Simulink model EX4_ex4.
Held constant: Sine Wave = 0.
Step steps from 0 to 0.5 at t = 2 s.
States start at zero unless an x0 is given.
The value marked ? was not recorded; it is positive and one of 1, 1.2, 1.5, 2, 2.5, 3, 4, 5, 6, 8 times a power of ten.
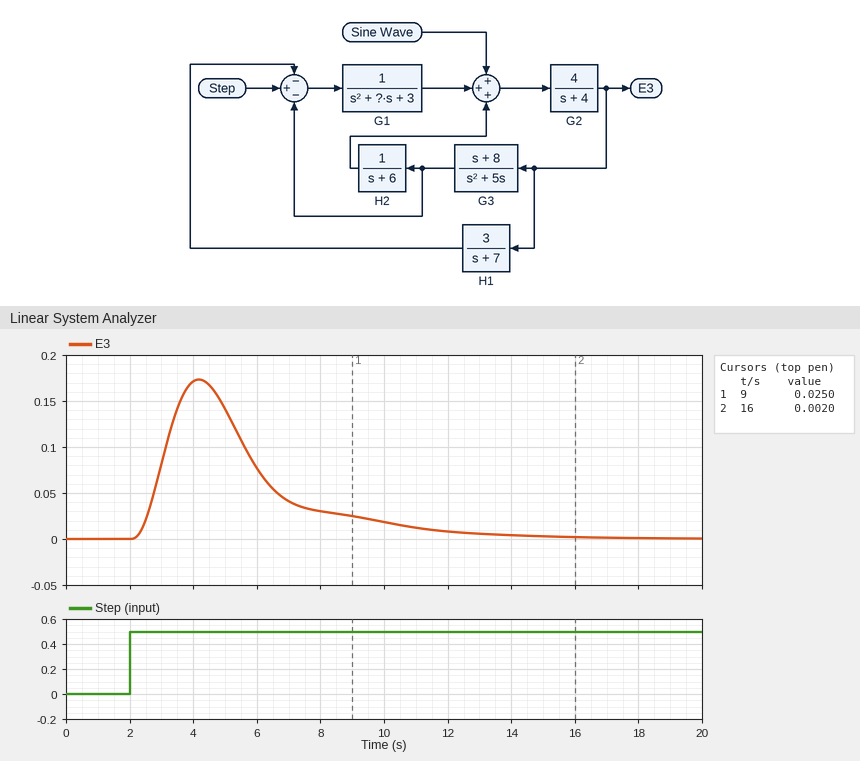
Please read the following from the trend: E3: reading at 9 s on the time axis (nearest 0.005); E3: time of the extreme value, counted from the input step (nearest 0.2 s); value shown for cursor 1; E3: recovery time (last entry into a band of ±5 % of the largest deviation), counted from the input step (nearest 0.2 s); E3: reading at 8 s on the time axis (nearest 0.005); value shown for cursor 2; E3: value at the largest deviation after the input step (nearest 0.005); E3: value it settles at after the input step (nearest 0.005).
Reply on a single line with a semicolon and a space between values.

0.025; 2.2 s; 0.0250; 9.8 s; 0.030; 0.0020; 0.175; 0.000
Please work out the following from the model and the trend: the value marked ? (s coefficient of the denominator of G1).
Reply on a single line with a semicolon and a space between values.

2
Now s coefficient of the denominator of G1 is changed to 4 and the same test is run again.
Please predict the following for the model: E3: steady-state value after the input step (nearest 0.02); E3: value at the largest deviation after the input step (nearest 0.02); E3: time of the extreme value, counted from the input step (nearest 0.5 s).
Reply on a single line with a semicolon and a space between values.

0.00; 0.14; 3.0 s
